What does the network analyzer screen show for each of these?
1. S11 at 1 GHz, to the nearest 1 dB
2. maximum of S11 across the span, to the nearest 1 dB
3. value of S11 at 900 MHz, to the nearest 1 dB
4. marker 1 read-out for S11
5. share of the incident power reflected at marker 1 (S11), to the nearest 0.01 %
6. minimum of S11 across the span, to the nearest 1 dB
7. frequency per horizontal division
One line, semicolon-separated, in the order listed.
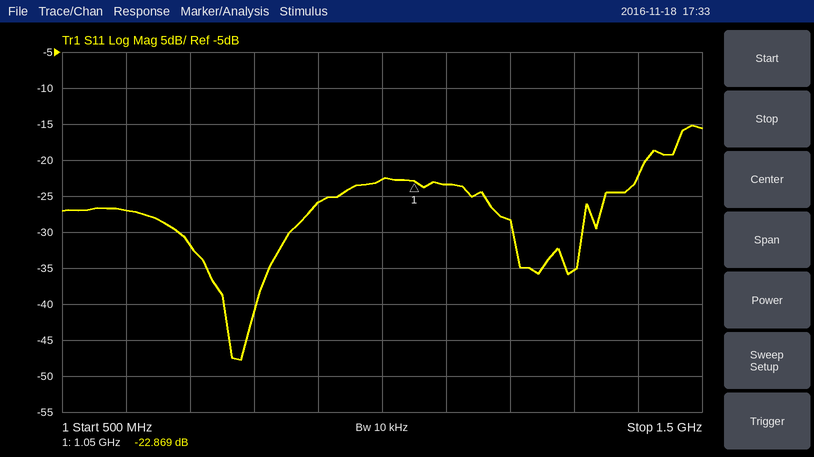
-23 dB; -15 dB; -26 dB; -22.869 dB; 0.52 %; -48 dB; 100 MHz
